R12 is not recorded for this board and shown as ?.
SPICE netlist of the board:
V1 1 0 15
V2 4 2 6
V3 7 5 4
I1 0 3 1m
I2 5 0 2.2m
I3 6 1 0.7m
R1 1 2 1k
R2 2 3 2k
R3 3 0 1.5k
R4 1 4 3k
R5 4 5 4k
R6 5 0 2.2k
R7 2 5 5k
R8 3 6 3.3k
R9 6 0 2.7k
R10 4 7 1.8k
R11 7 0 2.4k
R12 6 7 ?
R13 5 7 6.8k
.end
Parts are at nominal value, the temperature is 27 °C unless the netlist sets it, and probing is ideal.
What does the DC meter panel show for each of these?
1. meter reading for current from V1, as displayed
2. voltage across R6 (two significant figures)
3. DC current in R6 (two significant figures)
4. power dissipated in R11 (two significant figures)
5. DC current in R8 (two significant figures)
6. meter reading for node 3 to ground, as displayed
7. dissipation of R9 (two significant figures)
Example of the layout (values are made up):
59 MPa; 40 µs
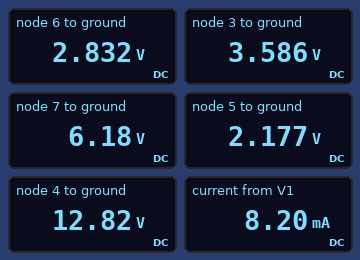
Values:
8.20 mA; 2.2 V; 990 µA; 16 mW; 230 µA; 3.586 V; 3.0 mW
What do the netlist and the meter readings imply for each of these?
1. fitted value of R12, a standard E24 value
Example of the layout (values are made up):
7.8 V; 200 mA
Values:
2.2 kΩ
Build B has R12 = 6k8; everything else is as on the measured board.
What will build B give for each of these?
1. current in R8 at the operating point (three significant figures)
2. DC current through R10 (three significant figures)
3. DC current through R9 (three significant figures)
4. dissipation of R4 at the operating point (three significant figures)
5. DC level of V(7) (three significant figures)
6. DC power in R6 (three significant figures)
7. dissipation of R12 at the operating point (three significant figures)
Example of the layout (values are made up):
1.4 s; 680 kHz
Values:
542 µA; 3.50 mA; 588 µA; 1.39 mW; 6.66 V; 3.22 mW; 3.79 mW
